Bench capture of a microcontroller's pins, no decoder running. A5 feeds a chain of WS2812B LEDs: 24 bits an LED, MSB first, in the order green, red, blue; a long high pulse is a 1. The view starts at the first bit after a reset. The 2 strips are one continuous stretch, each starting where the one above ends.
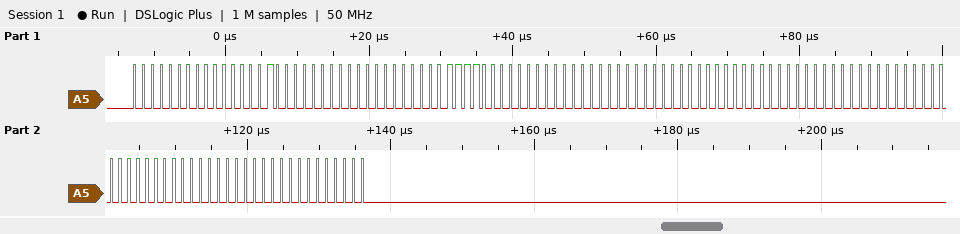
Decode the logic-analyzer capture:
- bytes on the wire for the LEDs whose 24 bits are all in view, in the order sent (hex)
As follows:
00 01 00 00 1E 00 00 00 00 00 00 00 00 00 00
